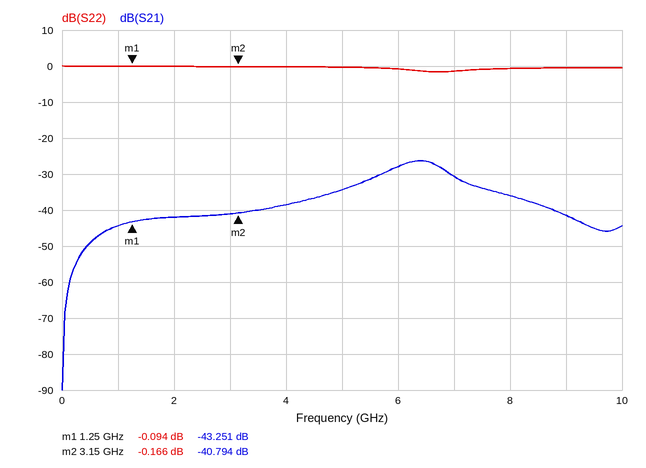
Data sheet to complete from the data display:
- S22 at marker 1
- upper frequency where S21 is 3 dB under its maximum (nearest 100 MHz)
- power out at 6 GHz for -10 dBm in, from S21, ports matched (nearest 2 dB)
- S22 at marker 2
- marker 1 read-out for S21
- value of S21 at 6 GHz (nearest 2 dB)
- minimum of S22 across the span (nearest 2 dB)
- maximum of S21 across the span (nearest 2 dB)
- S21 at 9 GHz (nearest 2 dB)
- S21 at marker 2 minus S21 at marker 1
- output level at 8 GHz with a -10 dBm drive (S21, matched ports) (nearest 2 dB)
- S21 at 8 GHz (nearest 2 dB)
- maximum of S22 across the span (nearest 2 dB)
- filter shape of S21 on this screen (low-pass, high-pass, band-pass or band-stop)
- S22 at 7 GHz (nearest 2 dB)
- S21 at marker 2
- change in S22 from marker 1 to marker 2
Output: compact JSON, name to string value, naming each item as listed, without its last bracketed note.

{"S22 at marker 1": "-0.094 dB", "upper frequency where S21 is 3 dB under its maximum": "6.9 GHz", "power out at 6 GHz for -10 dBm in, from S21, ports matched": "-38 dBm", "S22 at marker 2": "-0.166 dB", "marker 1 read-out for S21": "-43.251 dB", "value of S21 at 6 GHz": "-28 dB", "minimum of S22 across the span": "-2 dB", "maximum of S21 across the span": "-26 dB", "S21 at 9 GHz": "-42 dB", "S21 at marker 2 minus S21 at marker 1": "2.457 dB", "output level at 8 GHz with a -10 dBm drive (S21, matched ports)": "-46 dBm", "S21 at 8 GHz": "-36 dB", "maximum of S22 across the span": "0 dB", "filter shape of S21 on this screen": "band-pass", "S22 at 7 GHz": "-2 dB", "S21 at marker 2": "-40.794 dB", "change in S22 from marker 1 to marker 2": "-0.072 dB"}
